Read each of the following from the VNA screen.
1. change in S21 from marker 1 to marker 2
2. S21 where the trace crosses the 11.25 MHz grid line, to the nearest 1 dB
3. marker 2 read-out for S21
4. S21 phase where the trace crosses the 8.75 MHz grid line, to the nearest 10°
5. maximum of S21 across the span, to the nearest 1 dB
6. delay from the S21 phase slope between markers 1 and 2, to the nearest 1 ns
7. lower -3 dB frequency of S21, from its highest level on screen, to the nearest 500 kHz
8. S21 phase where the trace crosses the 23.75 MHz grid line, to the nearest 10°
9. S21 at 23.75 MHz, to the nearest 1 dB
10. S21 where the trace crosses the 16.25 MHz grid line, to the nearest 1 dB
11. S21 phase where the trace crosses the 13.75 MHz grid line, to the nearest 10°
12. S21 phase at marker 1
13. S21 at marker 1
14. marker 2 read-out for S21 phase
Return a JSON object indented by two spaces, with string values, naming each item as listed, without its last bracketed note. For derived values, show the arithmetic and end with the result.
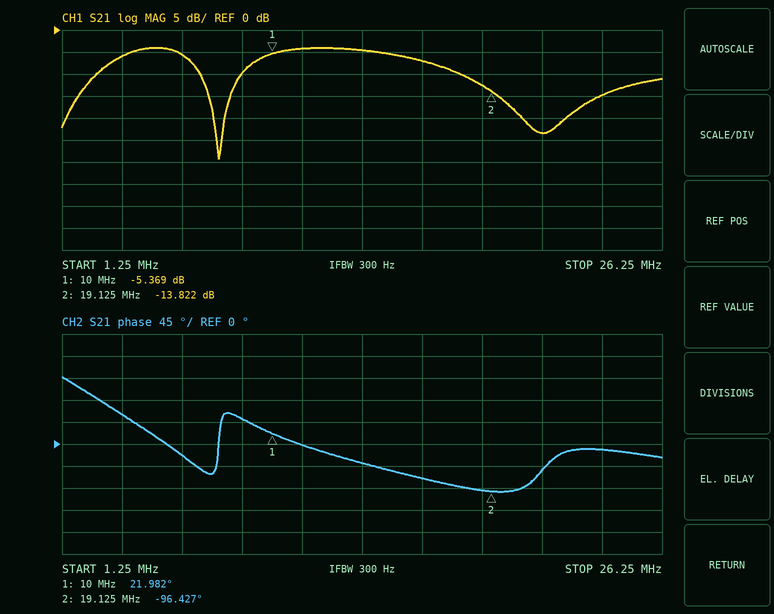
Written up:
{
  "change in S21 from marker 1 to marker 2": "-13.822 − (-5.369) = -8.453 dB",
  "S21 where the trace crosses the 11.25 MHz grid line, to the nearest 1 dB": "-4 dB",
  "marker 2 read-out for S21": "-13.822 dB",
  "S21 phase where the trace crosses the 8.75 MHz grid line, to the nearest 10°": "50°",
  "maximum of S21 across the span, to the nearest 1 dB": "-4 dB",
  "delay from the S21 phase slope between markers 1 and 2, to the nearest 1 ns": "−(-96.427° − (21.982°))/(360° × 9.125 MHz) ≈ 36 ns",
  "lower -3 dB frequency of S21, from its highest level on screen, to the nearest 500 kHz": "3.5 MHz",
  "S21 phase where the trace crosses the 23.75 MHz grid line, to the nearest 10°": "-10°",
  "S21 at 23.75 MHz, to the nearest 1 dB": "-15 dB",
  "S21 where the trace crosses the 16.25 MHz grid line, to the nearest 1 dB": "-7 dB",
  "S21 phase where the trace crosses the 13.75 MHz grid line, to the nearest 10°": "-40°",
  "S21 phase at marker 1": "21.982°",
  "S21 at marker 1": "-5.369 dB",
  "marker 2 read-out for S21 phase": "-96.427°"
}
